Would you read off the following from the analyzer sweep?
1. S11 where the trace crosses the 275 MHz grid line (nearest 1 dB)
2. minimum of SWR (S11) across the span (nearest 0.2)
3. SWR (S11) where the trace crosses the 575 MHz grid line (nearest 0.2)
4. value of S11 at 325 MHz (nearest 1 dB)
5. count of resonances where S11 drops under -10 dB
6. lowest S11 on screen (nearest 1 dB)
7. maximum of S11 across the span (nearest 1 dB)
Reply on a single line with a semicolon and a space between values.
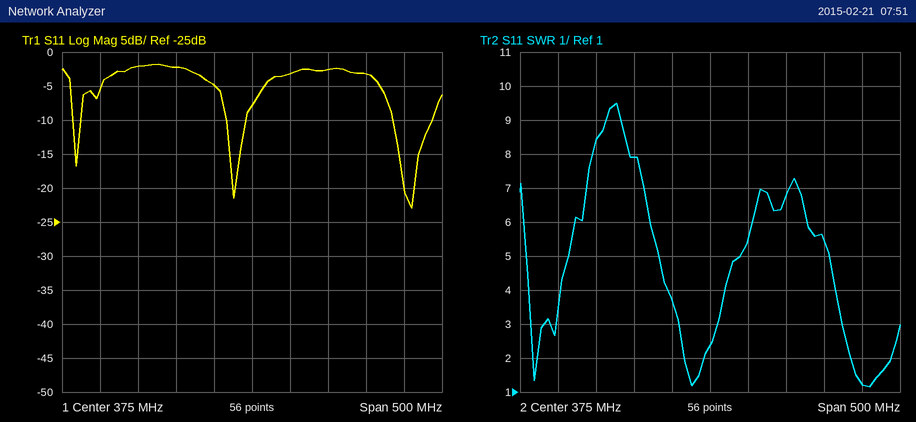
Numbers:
-2 dB; 1.2; 1.2; -5 dB; 3; -23 dB; -2 dB
